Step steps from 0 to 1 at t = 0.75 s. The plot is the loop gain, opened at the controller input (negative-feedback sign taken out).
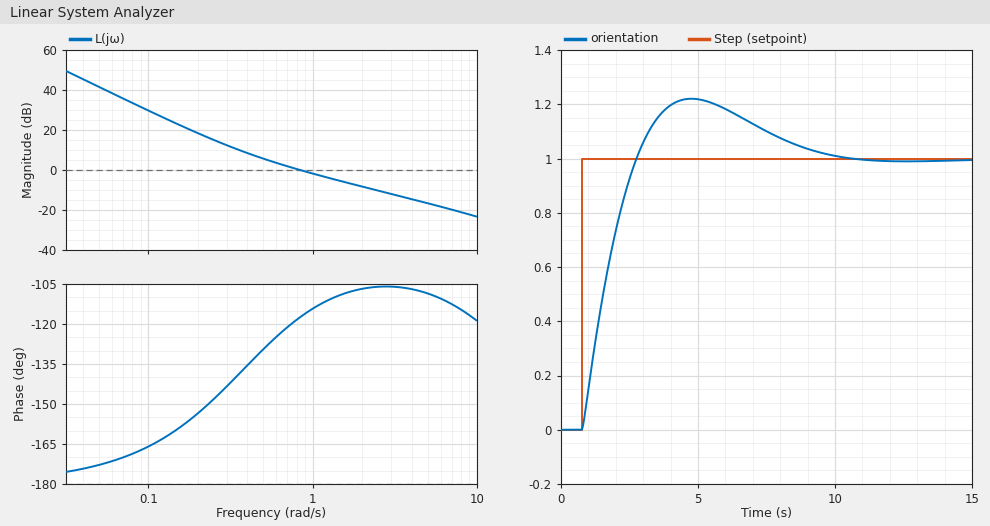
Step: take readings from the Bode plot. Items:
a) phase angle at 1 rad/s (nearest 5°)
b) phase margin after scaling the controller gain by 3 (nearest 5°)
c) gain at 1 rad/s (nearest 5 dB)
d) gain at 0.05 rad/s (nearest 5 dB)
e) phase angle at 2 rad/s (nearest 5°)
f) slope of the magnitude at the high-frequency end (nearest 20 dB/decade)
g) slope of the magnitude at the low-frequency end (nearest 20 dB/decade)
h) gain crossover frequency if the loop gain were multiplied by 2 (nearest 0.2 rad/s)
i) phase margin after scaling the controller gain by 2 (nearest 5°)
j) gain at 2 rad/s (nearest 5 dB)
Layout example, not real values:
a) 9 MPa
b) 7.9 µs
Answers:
a) -115°
b) 75°
c) 0 dB
d) 40 dB
e) -105°
f) -20 dB/decade
g) -40 dB/decade
h) 1.6 rad/s
i) 70°
j) -10 dB
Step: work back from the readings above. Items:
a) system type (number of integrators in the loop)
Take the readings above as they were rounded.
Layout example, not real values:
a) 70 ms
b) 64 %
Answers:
a) 2
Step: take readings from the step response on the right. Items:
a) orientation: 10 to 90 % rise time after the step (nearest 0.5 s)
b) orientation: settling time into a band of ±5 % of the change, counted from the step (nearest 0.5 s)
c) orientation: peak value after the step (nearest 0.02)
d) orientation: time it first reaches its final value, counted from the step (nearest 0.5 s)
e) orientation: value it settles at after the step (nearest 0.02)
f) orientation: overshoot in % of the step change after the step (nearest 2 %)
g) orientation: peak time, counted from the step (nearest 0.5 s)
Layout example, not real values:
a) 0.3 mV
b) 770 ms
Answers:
a) 1.5 s
b) 8.0 s
c) 1.22
d) 2.0 s
e) 1.00
f) 22 %
g) 4.0 s
